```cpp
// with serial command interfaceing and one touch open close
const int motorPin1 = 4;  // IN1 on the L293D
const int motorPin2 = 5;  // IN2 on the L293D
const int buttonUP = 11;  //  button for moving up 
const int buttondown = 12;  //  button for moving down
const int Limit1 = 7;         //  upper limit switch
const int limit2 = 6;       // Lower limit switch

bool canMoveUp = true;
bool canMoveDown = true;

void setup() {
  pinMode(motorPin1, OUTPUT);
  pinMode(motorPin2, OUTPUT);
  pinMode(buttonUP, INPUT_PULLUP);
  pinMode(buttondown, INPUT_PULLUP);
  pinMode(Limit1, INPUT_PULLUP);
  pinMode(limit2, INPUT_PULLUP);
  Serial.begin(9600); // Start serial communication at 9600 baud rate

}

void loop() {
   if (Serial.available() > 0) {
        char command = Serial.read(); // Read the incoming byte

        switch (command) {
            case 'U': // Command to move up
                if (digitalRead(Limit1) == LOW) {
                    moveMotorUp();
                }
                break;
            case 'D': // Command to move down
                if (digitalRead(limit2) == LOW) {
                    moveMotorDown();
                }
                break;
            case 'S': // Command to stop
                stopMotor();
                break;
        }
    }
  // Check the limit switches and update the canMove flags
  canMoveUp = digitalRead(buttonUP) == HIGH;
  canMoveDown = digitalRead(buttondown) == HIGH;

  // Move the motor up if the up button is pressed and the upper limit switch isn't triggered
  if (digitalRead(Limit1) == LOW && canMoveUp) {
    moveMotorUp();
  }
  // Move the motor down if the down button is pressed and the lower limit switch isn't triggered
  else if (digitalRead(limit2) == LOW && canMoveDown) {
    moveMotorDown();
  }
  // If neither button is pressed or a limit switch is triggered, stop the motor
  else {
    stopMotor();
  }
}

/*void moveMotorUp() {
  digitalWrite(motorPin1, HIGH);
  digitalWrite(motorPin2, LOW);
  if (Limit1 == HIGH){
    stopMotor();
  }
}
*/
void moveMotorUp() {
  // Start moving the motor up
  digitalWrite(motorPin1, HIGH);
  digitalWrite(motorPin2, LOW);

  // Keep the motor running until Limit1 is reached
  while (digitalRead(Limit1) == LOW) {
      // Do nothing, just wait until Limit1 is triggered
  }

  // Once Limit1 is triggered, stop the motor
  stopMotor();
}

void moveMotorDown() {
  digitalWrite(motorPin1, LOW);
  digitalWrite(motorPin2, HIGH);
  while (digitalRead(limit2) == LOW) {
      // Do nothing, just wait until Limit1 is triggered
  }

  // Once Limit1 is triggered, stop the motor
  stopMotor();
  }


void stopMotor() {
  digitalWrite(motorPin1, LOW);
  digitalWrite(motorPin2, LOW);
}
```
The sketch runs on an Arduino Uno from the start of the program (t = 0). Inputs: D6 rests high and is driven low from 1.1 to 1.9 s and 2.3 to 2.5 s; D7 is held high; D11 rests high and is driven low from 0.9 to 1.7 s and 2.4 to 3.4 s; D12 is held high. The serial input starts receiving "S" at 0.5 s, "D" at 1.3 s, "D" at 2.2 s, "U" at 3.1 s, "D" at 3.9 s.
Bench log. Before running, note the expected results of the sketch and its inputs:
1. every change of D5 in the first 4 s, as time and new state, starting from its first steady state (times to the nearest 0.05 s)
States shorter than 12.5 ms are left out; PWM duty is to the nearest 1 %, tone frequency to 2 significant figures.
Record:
0 s low; 1.1 s high; 1.9 s low; 2.3 s high; 2.5 s low
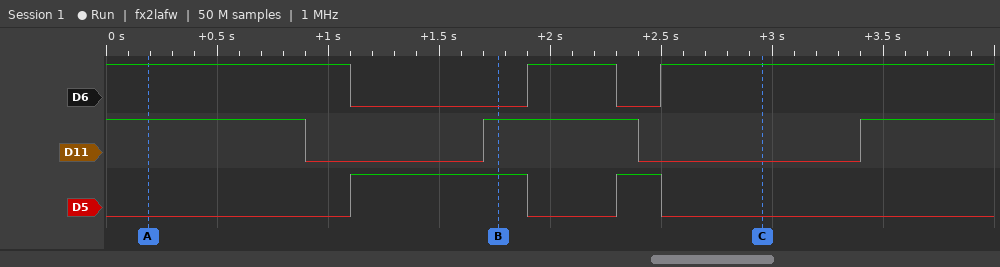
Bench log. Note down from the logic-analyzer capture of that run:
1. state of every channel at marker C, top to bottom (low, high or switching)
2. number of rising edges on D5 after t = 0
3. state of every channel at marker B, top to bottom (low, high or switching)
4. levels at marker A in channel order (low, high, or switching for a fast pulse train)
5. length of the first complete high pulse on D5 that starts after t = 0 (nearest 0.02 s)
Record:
D6 high, D11 low, D5 low
2
D6 low, D11 high, D5 high
D6 high, D11 high, D5 low
0.80 s
